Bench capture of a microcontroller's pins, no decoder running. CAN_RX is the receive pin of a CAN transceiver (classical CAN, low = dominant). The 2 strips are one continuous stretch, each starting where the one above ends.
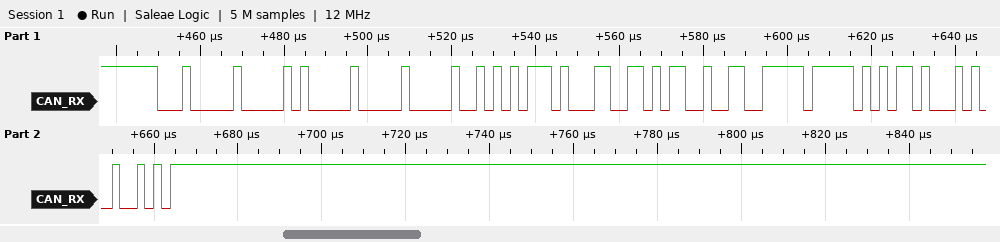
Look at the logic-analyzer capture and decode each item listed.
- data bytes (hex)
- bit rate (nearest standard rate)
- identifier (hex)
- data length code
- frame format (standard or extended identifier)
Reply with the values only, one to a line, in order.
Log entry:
00 02 AE 8C D6 4C FF EB
500 kbit/s
0x100
8
standard
